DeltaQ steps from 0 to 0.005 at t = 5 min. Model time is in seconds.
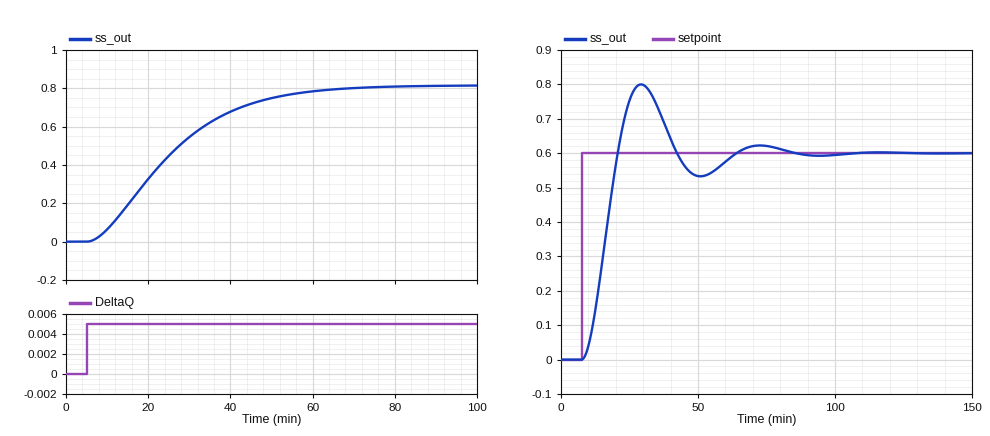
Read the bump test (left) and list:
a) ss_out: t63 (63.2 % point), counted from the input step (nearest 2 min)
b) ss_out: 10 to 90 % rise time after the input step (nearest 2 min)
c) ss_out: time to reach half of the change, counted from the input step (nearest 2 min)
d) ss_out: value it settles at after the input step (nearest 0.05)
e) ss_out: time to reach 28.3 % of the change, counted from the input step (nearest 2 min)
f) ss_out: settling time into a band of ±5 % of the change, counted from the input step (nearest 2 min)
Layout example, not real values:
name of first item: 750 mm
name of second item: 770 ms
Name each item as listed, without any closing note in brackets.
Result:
ss_out: t63 (63.2 % point), counted from the input step: 24 min
ss_out: 10 to 90 % rise time after the input step: 36 min
ss_out: time to reach half of the change, counted from the input step: 18 min
ss_out: value it settles at after the input step: 0.80
ss_out: time to reach 28.3 % of the change, counted from the input step: 12 min
ss_out: settling time into a band of ±5 % of the change, counted from the input step: 52 min
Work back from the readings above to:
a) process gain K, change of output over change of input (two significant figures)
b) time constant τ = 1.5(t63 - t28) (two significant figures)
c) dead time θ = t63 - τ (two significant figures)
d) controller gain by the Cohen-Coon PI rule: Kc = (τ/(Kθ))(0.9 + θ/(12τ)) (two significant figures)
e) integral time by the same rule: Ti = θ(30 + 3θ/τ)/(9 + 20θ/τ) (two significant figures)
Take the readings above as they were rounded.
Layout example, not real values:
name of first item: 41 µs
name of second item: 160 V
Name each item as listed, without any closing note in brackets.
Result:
process gain K, change of output over change of input: 160
time constant τ = 1.5(t63 - t28): 18 min
dead time θ = t63 - τ: 6.0 min
controller gain by the Cohen-Coon PI rule: Kc = (τ/(Kθ))(0.9 + θ/(12τ)): 0.017
integral time by the same rule: Ti = θ(30 + 3θ/τ)/(9 + 20θ/τ): 12 min
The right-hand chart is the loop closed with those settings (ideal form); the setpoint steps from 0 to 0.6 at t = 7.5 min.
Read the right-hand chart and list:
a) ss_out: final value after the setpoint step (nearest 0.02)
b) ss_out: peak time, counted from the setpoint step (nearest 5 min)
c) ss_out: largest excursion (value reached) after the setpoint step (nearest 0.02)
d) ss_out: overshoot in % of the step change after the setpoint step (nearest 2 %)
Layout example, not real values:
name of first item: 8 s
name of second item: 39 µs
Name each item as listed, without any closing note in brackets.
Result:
ss_out: final value after the setpoint step: 0.60
ss_out: peak time, counted from the setpoint step: 20 min
ss_out: largest excursion (value reached) after the setpoint step: 0.80
ss_out: overshoot in % of the step change after the setpoint step: 34 %
